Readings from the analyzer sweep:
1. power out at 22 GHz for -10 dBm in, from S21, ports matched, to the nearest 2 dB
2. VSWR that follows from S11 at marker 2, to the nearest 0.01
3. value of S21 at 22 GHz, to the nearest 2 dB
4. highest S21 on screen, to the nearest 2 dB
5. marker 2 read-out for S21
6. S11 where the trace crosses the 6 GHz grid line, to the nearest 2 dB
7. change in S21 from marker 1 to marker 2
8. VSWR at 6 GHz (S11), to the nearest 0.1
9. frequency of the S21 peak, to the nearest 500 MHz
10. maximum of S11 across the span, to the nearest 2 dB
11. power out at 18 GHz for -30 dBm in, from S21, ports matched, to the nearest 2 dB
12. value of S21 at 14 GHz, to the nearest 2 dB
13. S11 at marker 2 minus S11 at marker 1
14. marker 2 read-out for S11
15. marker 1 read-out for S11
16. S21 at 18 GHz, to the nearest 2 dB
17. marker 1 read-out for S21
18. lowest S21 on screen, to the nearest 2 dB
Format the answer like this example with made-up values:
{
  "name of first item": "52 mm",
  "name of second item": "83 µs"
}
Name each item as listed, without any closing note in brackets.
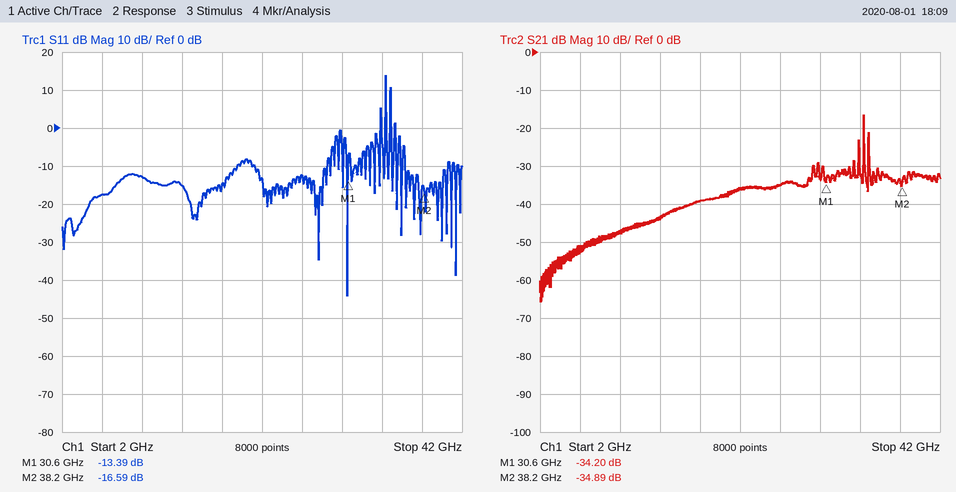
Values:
{
  "power out at 22 GHz for -10 dBm in, from S21, ports matched, to the nearest 2 dB": "-46 dBm",
  "VSWR that follows from S11 at marker 2, to the nearest 0.01": "1.35",
  "value of S21 at 22 GHz, to the nearest 2 dB": "-36 dB",
  "highest S21 on screen, to the nearest 2 dB": "-16 dB",
  "marker 2 read-out for S21": "-34.89 dB",
  "S11 where the trace crosses the 6 GHz grid line, to the nearest 2 dB": "-18 dB",
  "change in S21 from marker 1 to marker 2": "-0.69 dB",
  "VSWR at 6 GHz (S11), to the nearest 0.1": "1.3",
  "frequency of the S21 peak, to the nearest 500 MHz": "34.5 GHz",
  "maximum of S11 across the span, to the nearest 2 dB": "14 dB",
  "power out at 18 GHz for -30 dBm in, from S21, ports matched, to the nearest 2 dB": "-70 dBm",
  "value of S21 at 14 GHz, to the nearest 2 dB": "-44 dB",
  "S11 at marker 2 minus S11 at marker 1": "-3.20 dB",
  "marker 2 read-out for S11": "-16.59 dB",
  "marker 1 read-out for S11": "-13.39 dB",
  "S21 at 18 GHz, to the nearest 2 dB": "-40 dB",
  "marker 1 read-out for S21": "-34.20 dB",
  "lowest S21 on screen, to the nearest 2 dB": "-66 dB"
}
